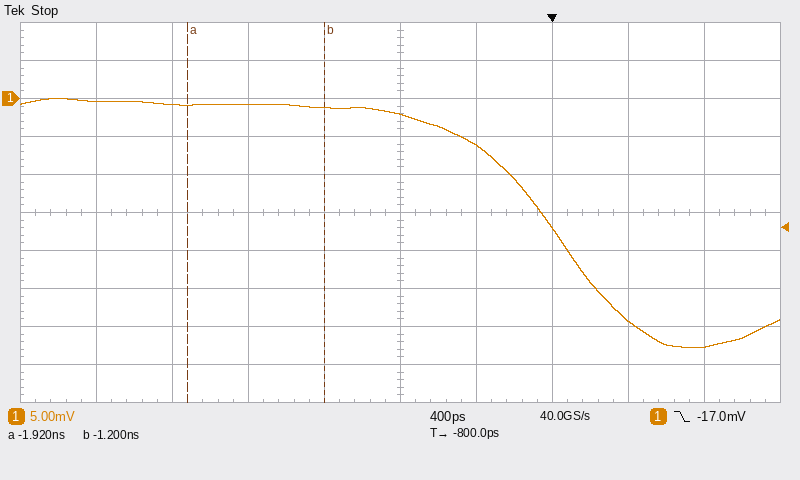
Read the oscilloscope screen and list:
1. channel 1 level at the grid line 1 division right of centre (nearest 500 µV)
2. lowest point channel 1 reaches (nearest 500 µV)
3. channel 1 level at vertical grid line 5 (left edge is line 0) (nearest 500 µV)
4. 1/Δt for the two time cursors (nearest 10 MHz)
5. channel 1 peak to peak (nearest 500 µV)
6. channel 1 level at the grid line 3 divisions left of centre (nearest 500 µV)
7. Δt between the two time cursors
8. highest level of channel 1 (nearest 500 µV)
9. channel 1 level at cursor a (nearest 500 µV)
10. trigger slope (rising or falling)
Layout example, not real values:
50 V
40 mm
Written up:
-6.0 mV
-33.0 mV
-2.0 mV
1.39 GHz
33.0 mV
-1.0 mV
720 ps
0.0 mV
-1.0 mV
falling
